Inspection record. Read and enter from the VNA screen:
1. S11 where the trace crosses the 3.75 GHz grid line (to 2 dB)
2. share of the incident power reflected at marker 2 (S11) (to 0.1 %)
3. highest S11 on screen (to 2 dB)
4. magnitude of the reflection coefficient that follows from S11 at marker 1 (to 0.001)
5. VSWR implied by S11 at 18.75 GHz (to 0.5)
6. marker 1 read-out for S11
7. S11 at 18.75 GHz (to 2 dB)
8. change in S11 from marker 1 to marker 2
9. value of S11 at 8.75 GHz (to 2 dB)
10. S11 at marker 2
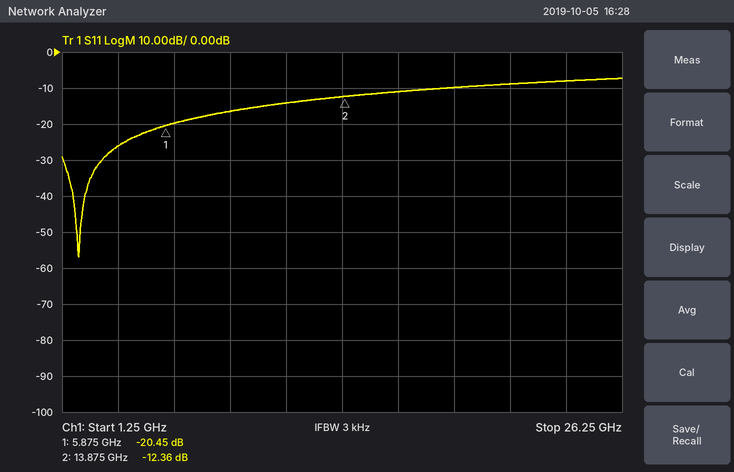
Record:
-26 dB
5.8 %
-8 dB
0.095
2.0
-20.45 dB
-10 dB
8.09 dB
-16 dB
-12.36 dB
